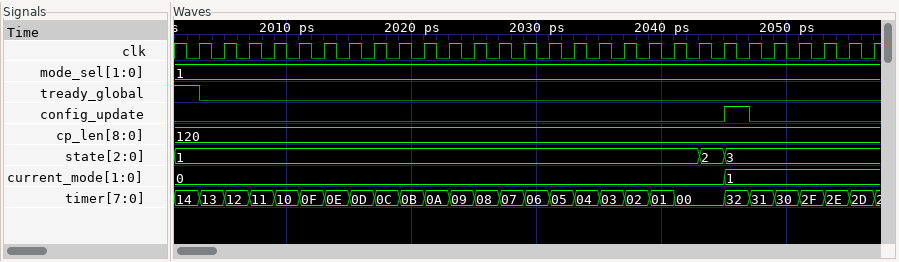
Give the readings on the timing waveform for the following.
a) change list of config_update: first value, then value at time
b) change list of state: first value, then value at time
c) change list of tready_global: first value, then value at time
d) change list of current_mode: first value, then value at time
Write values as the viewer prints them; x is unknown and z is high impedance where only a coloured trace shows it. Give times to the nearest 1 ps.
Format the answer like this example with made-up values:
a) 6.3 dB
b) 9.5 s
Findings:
a) 0, 1 at 2045 ps, 0 at 2047 ps
b) 1, 2 at 2043 ps, 3 at 2045 ps
c) 1, 0 at 2003 ps
d) 0, 1 at 2045 ps
